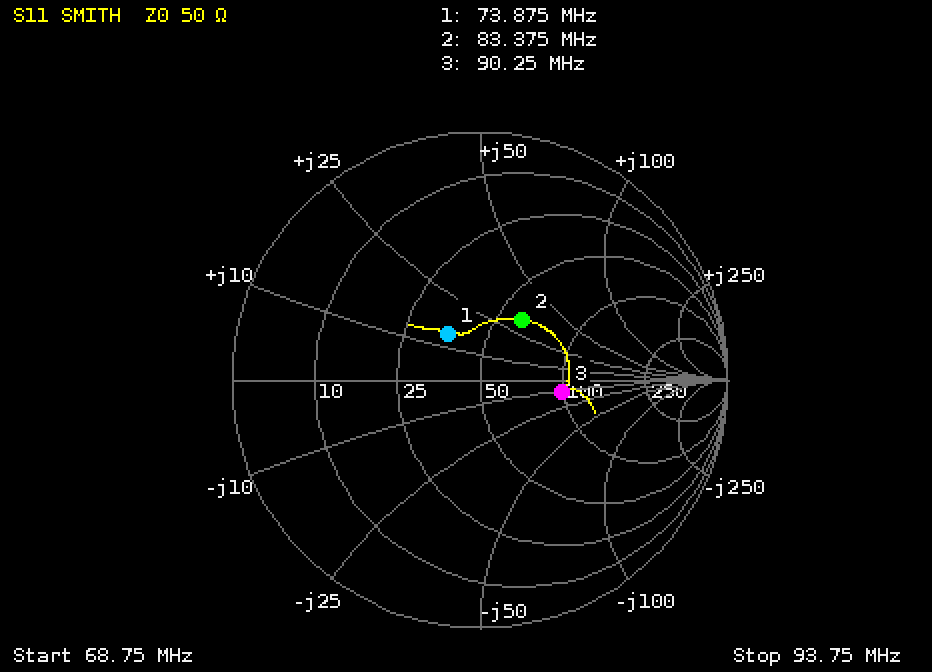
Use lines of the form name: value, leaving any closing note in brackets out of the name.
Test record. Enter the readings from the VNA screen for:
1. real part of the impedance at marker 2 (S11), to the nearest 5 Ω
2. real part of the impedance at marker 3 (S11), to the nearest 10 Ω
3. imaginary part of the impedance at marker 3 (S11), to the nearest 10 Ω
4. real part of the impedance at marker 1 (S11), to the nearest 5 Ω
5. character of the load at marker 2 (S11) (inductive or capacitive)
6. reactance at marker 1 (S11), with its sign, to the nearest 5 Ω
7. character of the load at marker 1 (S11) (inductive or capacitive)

real part of the impedance at marker 2 (S11), to the nearest 5 Ω: 60 Ω
real part of the impedance at marker 3 (S11), to the nearest 10 Ω: 100 Ω
imaginary part of the impedance at marker 3 (S11), to the nearest 10 Ω: -10 Ω
real part of the impedance at marker 1 (S11), to the nearest 5 Ω: 35 Ω
character of the load at marker 2 (S11): inductive
reactance at marker 1 (S11), with its sign, to the nearest 5 Ω: +15 Ω
character of the load at marker 1 (S11): inductive
